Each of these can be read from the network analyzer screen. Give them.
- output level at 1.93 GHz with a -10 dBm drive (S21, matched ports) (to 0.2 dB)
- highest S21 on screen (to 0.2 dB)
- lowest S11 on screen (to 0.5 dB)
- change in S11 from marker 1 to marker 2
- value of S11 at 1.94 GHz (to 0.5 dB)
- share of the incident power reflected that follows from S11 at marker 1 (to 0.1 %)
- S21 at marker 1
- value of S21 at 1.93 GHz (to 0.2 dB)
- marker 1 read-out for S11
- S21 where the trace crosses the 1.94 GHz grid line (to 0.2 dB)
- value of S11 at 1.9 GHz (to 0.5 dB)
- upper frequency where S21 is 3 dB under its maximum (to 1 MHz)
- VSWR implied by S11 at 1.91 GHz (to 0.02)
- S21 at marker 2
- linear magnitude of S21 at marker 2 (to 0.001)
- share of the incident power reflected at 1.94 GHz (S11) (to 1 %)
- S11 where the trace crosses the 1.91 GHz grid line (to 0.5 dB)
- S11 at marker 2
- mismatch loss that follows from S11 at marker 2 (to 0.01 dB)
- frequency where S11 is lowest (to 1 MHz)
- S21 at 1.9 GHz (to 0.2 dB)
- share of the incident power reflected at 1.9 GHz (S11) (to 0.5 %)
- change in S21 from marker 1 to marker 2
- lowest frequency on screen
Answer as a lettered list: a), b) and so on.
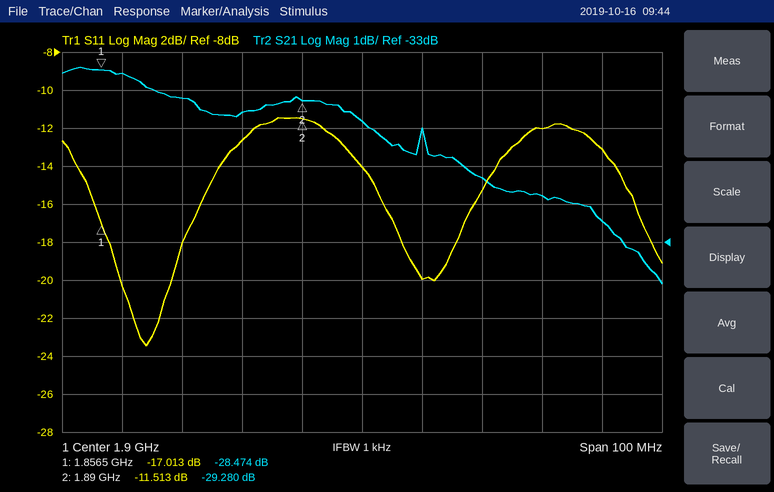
a) -41.8 dBm
b) -28.4 dB
c) -23.5 dB
d) 5.500 dB
e) -13.0 dB
f) 2.0 %
g) -28.474 dB
h) -31.8 dB
i) -17.013 dB
j) -32.4 dB
k) -14.0 dB
l) 1.921 GHz
m) 1.22
n) -29.280 dB
o) 0.034
p) 5 %
q) -20.0 dB
r) -11.513 dB
s) 0.32 dB
t) 1.864 GHz
u) -29.8 dB
v) 4.0 %
w) -0.806 dB
x) 1.85 GHz
